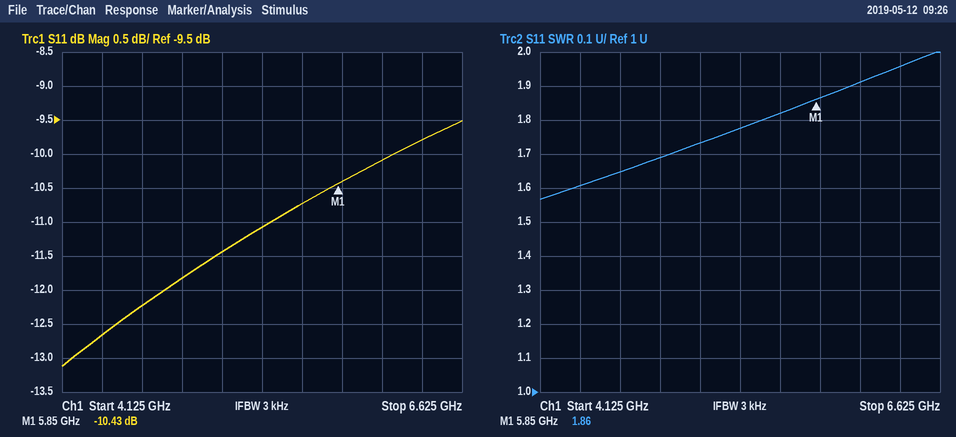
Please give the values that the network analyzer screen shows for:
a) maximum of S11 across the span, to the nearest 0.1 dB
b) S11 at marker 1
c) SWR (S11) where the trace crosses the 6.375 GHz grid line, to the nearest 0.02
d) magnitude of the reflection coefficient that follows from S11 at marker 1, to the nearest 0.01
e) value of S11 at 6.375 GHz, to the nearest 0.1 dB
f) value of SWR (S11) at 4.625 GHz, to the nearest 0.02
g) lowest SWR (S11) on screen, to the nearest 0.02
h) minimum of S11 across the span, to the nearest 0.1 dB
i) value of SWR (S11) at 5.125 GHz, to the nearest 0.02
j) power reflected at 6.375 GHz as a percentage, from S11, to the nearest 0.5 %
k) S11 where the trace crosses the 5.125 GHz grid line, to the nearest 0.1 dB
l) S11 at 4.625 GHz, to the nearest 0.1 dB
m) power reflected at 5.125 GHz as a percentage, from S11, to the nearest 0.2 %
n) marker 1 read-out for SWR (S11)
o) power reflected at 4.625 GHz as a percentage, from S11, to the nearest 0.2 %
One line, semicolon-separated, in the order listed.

-9.5 dB; -10.43 dB; 1.96; 0.30; -9.8 dB; 1.64; 1.56; -13.1 dB; 1.74; 10.5 %; -11.4 dB; -12.2 dB; 7.2 %; 1.86; 6.0 %
